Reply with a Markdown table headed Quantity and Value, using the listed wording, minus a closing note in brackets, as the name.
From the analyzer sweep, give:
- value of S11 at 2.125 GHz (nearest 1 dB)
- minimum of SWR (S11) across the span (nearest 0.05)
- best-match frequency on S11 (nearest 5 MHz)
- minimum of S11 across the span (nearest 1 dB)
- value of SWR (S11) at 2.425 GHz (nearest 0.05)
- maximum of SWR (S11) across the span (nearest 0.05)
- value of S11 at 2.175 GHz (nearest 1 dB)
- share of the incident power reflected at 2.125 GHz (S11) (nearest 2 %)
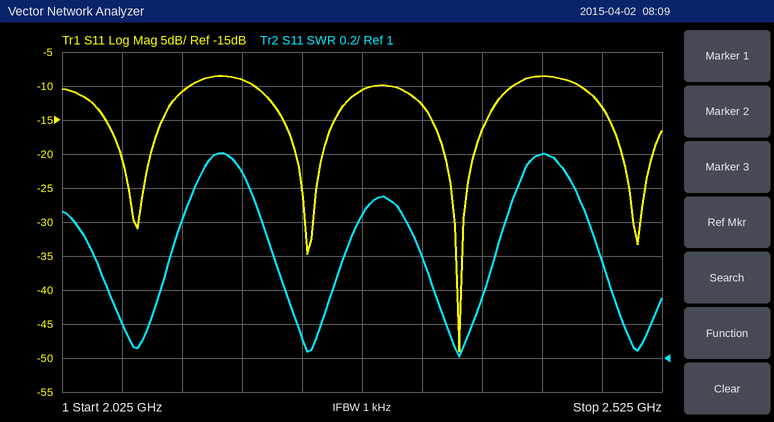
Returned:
| Quantity | Value |
|---|---|
| value of S11 at 2.125 GHz | -11 dB |
| minimum of SWR (S11) across the span | 1.00 |
| best-match frequency on S11 | 2.355 GHz |
| minimum of S11 across the span | -49 dB |
| value of SWR (S11) at 2.425 GHz | 2.20 |
| maximum of SWR (S11) across the span | 2.20 |
| value of S11 at 2.175 GHz | -9 dB |
| share of the incident power reflected at 2.125 GHz (S11) | 8 % |
